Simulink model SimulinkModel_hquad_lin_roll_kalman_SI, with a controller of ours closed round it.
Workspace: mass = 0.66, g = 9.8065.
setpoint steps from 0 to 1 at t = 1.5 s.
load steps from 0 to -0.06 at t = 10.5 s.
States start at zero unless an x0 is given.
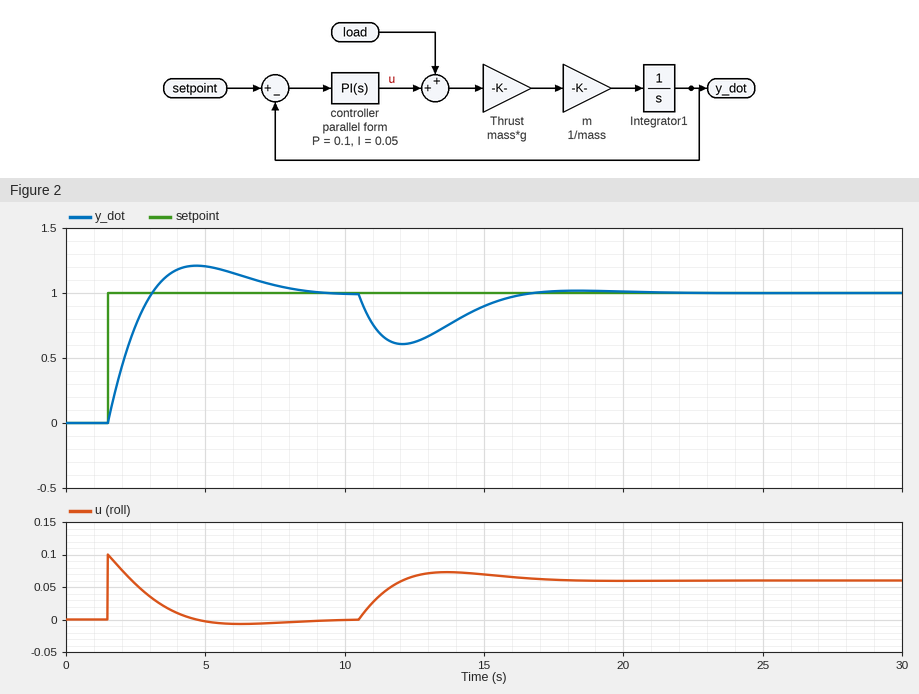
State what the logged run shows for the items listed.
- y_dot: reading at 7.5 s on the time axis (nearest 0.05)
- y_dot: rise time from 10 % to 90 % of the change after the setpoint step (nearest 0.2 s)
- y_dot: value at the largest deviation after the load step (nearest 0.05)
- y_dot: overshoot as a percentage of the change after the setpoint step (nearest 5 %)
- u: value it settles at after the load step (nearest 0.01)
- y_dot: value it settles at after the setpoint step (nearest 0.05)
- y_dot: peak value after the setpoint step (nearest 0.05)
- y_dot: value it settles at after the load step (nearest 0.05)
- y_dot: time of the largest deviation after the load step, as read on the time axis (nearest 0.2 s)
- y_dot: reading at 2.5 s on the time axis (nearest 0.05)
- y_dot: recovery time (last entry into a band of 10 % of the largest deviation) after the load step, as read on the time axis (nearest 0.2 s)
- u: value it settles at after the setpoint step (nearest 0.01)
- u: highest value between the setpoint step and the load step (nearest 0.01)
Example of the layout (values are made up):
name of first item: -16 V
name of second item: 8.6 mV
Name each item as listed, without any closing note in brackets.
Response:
y_dot: reading at 7.5 s on the time axis: 1.05
y_dot: rise time from 10 % to 90 % of the change after the setpoint step: 1.2 s
y_dot: value at the largest deviation after the load step: 0.60
y_dot: overshoot as a percentage of the change after the setpoint step: 20 %
u: value it settles at after the load step: 0.06
y_dot: value it settles at after the setpoint step: 1.00
y_dot: peak value after the setpoint step: 1.20
y_dot: value it settles at after the load step: 1.00
y_dot: time of the largest deviation after the load step, as read on the time axis: 12.0 s
y_dot: reading at 2.5 s on the time axis: 0.75
y_dot: recovery time (last entry into a band of 10 % of the largest deviation) after the load step, as read on the time axis: 15.8 s
u: value it settles at after the setpoint step: 0.00
u: highest value between the setpoint step and the load step: 0.10
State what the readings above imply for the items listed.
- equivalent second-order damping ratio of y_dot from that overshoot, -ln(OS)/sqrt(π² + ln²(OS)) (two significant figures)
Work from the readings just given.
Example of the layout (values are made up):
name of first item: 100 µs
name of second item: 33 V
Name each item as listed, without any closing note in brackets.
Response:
equivalent second-order damping ratio of y_dot from that overshoot, -ln(OS)/sqrt(π² + ln²(OS)): 0.46
